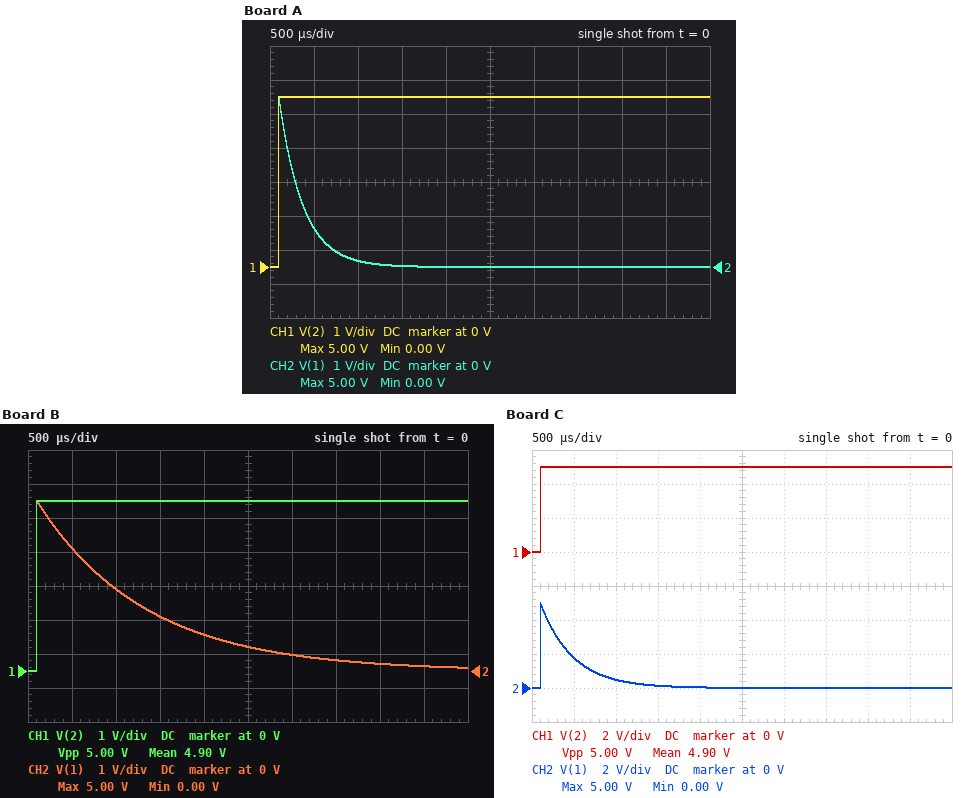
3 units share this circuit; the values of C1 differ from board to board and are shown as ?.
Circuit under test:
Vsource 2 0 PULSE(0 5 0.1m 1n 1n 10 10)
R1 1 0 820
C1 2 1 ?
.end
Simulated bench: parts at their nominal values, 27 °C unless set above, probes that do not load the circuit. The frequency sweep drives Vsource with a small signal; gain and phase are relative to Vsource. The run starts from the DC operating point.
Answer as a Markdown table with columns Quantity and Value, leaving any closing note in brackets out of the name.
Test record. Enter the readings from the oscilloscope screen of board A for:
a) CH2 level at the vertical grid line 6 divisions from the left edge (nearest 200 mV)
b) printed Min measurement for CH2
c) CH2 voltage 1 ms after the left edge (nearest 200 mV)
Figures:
| Quantity | Value |
|---|---|
| CH2 level at the vertical grid line 6 divisions from the left edge | 0 V |
| printed Min measurement for CH2 | 0.00 V |
| CH2 voltage 1 ms after the left edge | 200 mV |
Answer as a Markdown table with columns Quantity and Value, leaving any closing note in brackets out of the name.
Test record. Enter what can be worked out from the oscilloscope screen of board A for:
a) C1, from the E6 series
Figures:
| Quantity | Value |
|---|---|
| C1, from the E6 series | 330 nF |
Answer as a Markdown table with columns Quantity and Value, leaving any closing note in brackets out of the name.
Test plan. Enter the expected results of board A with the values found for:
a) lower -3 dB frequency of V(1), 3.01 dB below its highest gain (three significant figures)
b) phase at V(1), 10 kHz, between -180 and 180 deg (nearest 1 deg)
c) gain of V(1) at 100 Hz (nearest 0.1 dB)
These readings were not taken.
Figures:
| Quantity | Value |
|---|---|
| lower -3 dB frequency of V(1), 3.01 dB below its highest gain | 588 Hz |
| phase at V(1), 10 kHz, between -180 and 180 deg | 3 deg |
| gain of V(1) at 100 Hz | -15.5 dB |
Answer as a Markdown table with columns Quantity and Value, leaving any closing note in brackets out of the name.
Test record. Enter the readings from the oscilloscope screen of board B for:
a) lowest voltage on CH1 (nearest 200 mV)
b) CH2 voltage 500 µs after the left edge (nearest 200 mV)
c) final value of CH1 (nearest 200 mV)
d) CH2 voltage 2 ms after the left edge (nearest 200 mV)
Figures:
| Quantity | Value |
|---|---|
| lowest voltage on CH1 | 0 V |
| CH2 voltage 500 µs after the left edge | 3.6 V |
| final value of CH1 | 5.0 V |
| CH2 voltage 2 ms after the left edge | 1.0 V |
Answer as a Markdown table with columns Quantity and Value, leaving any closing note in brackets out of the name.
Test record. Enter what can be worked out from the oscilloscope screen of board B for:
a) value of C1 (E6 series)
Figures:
| Quantity | Value |
|---|---|
| value of C1 | 1.5 µF |
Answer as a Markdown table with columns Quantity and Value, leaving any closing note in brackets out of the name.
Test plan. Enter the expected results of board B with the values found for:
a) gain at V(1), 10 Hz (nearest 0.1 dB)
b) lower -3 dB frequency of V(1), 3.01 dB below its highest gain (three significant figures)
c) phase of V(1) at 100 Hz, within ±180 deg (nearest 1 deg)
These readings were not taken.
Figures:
| Quantity | Value |
|---|---|
| gain at V(1), 10 Hz | -22.3 dB |
| lower -3 dB frequency of V(1), 3.01 dB below its highest gain | 129 Hz |
| phase of V(1) at 100 Hz, within ±180 deg | 52 deg |
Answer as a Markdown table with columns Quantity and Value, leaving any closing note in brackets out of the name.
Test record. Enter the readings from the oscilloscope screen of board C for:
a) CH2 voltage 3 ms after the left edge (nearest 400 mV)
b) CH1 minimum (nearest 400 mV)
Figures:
| Quantity | Value |
|---|---|
| CH2 voltage 3 ms after the left edge | 0 V |
| CH1 minimum | 0 V |
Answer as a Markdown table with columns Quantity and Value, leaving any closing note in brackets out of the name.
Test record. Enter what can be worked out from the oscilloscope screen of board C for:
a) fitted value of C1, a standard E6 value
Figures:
| Quantity | Value |
|---|---|
| fitted value of C1, a standard E6 value | 470 nF |
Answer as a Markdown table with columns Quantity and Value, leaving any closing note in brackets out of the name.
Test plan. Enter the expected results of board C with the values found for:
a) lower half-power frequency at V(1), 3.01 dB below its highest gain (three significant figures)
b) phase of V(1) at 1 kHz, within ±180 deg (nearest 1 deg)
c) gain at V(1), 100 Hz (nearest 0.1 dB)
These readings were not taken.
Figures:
| Quantity | Value |
|---|---|
| lower half-power frequency at V(1), 3.01 dB below its highest gain | 413 Hz |
| phase of V(1) at 1 kHz, within ±180 deg | 22 deg |
| gain at V(1), 100 Hz | -12.6 dB |
